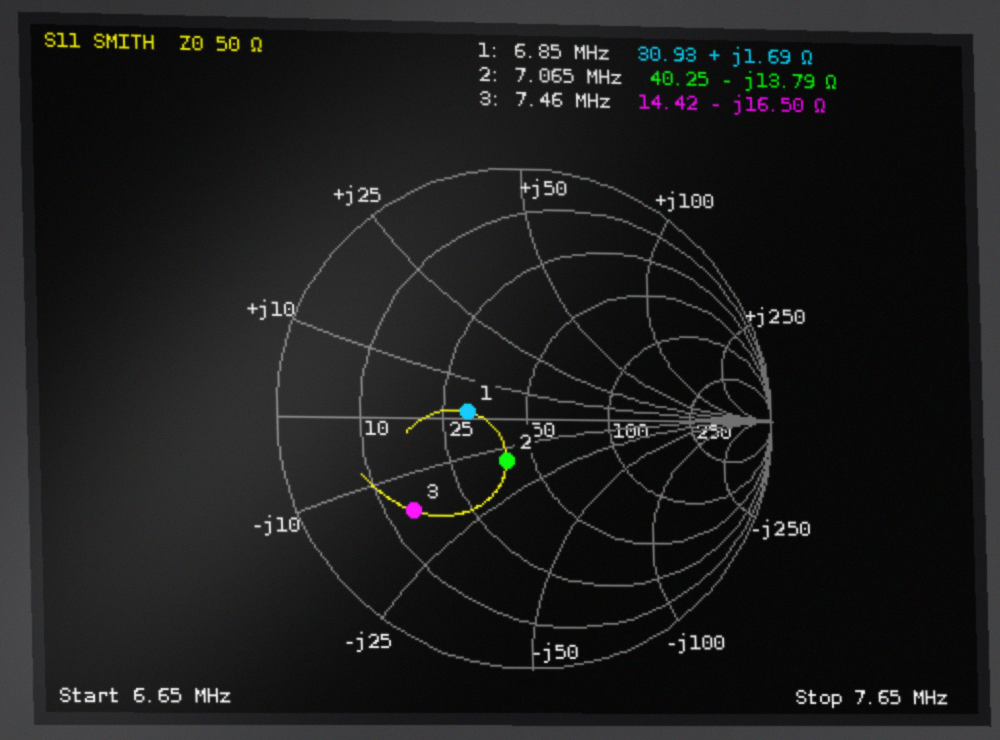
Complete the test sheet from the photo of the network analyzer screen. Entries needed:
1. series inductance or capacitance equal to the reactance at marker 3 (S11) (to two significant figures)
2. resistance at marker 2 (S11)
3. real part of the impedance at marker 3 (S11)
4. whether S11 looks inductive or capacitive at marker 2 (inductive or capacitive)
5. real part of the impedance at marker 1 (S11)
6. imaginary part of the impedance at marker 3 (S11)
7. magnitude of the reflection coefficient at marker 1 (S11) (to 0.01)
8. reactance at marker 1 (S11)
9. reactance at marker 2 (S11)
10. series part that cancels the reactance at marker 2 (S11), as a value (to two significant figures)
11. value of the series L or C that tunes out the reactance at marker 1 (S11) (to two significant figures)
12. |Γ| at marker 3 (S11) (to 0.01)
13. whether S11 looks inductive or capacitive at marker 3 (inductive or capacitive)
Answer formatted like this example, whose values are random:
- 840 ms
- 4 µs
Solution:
- 1.3 nF
- 40.25 Ω
- 14.42 Ω
- capacitive
- 30.93 Ω
- -16.50 Ω
- 0.24
- +1.69 Ω
- -13.79 Ω
- 310 nH
- 14 nF
- 0.59
- capacitive
